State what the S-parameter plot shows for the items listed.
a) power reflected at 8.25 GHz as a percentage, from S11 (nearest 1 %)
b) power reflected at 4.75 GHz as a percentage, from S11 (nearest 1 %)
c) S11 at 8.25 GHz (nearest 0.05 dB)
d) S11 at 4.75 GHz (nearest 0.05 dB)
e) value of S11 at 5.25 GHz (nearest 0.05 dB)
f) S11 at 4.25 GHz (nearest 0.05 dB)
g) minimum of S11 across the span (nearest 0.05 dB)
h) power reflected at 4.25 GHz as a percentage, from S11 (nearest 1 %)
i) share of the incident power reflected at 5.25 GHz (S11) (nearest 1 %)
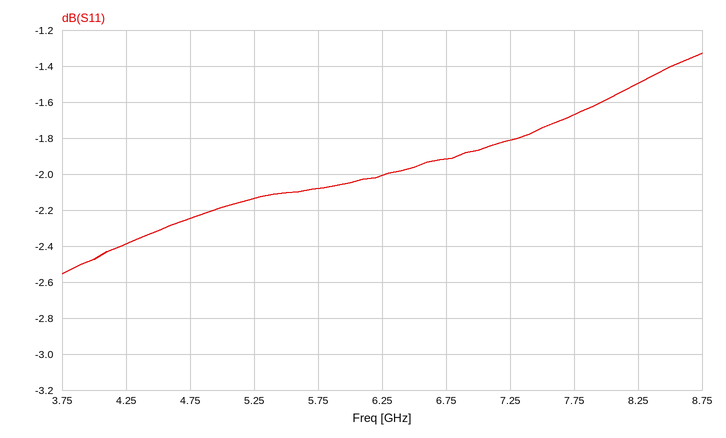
71 %
60 %
-1.50 dB
-2.25 dB
-2.15 dB
-2.40 dB
-2.55 dB
58 %
61 %
